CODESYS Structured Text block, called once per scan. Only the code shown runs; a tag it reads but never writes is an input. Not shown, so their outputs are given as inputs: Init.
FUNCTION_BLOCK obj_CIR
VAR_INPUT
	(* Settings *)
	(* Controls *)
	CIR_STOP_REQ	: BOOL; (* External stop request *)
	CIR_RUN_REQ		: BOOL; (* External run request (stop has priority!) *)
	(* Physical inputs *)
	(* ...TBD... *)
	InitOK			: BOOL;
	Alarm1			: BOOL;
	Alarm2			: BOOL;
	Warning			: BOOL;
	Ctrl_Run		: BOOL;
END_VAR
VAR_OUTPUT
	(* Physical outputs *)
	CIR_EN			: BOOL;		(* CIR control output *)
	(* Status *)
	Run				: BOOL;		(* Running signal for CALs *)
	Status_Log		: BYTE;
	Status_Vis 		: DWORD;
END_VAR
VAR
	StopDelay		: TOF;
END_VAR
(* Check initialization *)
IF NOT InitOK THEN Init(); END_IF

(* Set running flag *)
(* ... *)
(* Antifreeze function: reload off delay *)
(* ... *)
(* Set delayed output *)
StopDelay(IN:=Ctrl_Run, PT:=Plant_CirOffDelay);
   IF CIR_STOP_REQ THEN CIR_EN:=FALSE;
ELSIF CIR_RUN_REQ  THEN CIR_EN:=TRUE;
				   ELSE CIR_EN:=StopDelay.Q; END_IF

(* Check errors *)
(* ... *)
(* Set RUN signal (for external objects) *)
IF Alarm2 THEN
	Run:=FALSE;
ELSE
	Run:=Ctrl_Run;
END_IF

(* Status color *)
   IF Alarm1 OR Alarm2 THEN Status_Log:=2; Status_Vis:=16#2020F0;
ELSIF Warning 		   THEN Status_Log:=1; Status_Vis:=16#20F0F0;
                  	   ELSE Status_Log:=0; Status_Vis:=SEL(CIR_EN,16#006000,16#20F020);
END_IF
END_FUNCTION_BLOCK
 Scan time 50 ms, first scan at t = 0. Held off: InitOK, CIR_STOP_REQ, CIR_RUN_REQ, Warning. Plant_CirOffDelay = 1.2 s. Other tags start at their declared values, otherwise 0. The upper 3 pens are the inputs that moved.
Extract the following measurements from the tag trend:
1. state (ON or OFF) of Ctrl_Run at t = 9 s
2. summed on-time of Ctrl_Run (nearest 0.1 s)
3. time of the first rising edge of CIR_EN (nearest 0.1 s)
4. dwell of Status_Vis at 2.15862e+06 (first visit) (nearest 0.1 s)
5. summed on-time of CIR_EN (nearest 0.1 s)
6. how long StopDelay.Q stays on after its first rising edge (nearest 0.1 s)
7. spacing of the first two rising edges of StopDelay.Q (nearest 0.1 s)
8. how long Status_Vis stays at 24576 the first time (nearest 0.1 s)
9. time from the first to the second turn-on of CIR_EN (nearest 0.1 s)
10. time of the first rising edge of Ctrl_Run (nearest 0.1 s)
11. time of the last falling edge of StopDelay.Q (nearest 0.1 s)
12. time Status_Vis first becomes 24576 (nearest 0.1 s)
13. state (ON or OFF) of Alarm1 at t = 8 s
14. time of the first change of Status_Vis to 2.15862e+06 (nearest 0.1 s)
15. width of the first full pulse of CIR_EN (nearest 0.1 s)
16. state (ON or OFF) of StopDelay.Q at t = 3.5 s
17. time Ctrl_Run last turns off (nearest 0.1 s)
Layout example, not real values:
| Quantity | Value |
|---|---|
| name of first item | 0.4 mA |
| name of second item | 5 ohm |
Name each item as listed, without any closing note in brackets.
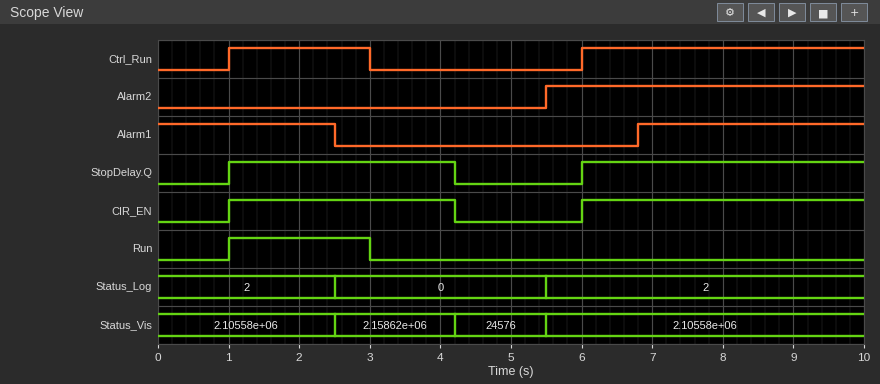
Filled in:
| Quantity | Value |
|---|---|
| state (ON or OFF) of Ctrl_Run at t = 9 s | ON |
| summed on-time of Ctrl_Run | 6.0 s |
| time of the first rising edge of CIR_EN | 1.0 s |
| dwell of Status_Vis at 2.15862e+06 (first visit) | 1.7 s |
| summed on-time of CIR_EN | 7.2 s |
| how long StopDelay.Q stays on after its first rising edge | 3.2 s |
| spacing of the first two rising edges of StopDelay.Q | 5.0 s |
| how long Status_Vis stays at 24576 the first time | 1.3 s |
| time from the first to the second turn-on of CIR_EN | 5.0 s |
| time of the first rising edge of Ctrl_Run | 1.0 s |
| time of the last falling edge of StopDelay.Q | 4.2 s |
| time Status_Vis first becomes 24576 | 4.2 s |
| state (ON or OFF) of Alarm1 at t = 8 s | ON |
| time of the first change of Status_Vis to 2.15862e+06 | 2.5 s |
| width of the first full pulse of CIR_EN | 3.2 s |
| state (ON or OFF) of StopDelay.Q at t = 3.5 s | ON |
| time Ctrl_Run last turns off | 3.0 s |
